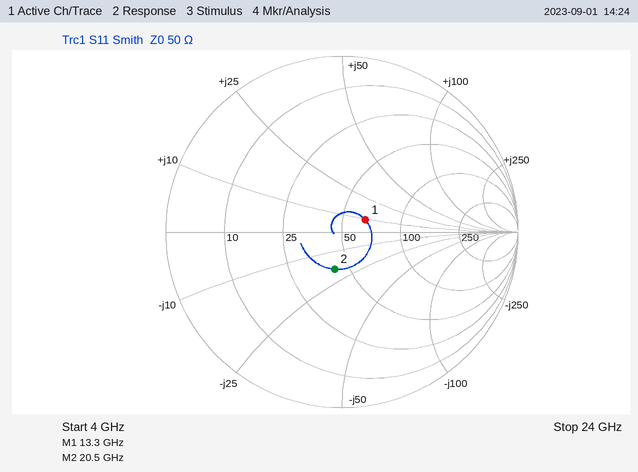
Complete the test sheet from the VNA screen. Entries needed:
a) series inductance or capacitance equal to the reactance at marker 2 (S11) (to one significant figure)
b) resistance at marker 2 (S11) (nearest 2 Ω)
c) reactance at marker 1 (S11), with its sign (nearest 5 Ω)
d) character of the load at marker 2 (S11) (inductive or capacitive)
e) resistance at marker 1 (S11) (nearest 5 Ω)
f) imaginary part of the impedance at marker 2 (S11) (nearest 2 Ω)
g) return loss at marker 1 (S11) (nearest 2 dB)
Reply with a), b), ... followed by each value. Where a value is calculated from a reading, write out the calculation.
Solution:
a) C = 1/(2π × 20.5 GHz × 18 Ω) ≈ 431 fF, so 400 fF to one significant figure
b) 42 Ω
c) +10 Ω
d) capacitive
e) 65 Ω
f) -18 Ω
g) 16 dB
